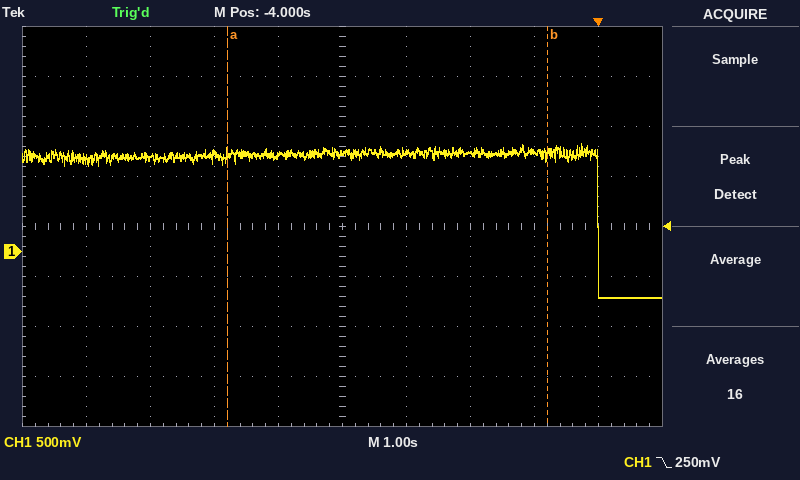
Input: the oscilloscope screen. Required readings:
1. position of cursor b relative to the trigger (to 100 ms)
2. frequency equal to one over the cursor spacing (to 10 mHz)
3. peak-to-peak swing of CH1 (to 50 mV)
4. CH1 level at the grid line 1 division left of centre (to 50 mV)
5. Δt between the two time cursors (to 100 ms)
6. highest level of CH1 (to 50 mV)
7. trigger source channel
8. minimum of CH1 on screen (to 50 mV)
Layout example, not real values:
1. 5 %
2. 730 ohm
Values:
1. -800 ms
2. 200 mHz
3. 1.55 V
4. 950 mV
5. 5.0 s
6. 1.10 V
7. CH1
8. -450 mV
